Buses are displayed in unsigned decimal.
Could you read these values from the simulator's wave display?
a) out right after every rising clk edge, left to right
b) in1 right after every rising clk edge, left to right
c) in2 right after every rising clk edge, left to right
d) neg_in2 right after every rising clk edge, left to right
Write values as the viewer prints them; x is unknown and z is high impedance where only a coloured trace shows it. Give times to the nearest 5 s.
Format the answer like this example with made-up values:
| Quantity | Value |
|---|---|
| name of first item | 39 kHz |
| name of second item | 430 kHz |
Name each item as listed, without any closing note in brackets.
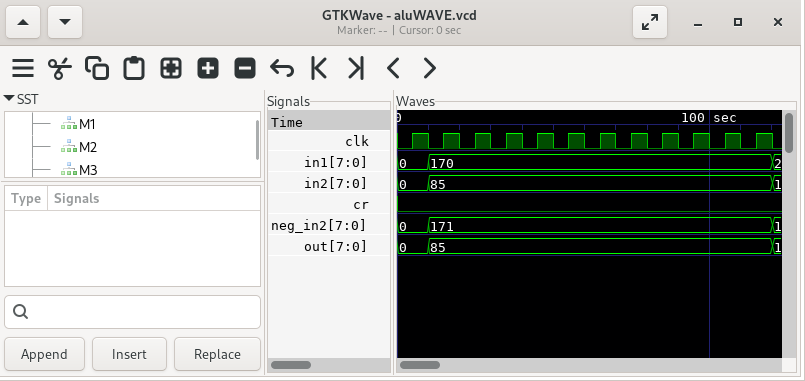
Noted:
| Quantity | Value |
|---|---|
| out right after every rising clk edge, left to right | 0, 85, 85, 85, 85, 85, 85, 85, 85, 85, 85, 85 |
| in1 right after every rising clk edge, left to right | 0, 170, 170, 170, 170, 170, 170, 170, 170, 170, 170, 170 |
| in2 right after every rising clk edge, left to right | 0, 85, 85, 85, 85, 85, 85, 85, 85, 85, 85, 85 |
| neg_in2 right after every rising clk edge, left to right | 0, 171, 171, 171, 171, 171, 171, 171, 171, 171, 171, 171 |
